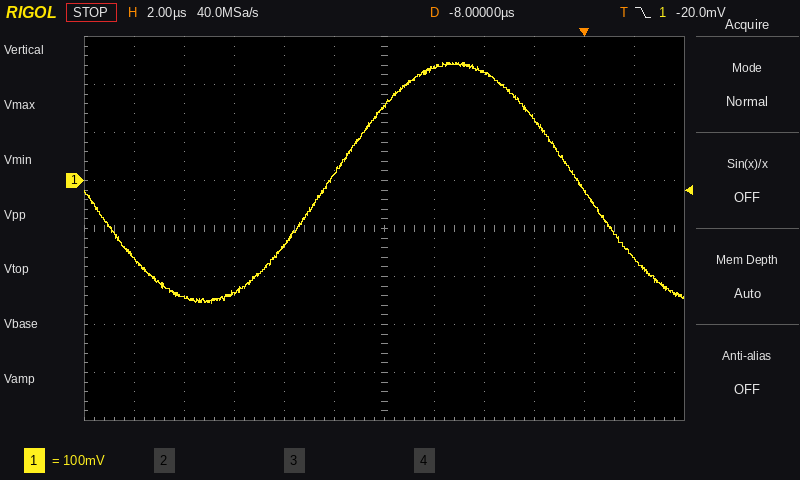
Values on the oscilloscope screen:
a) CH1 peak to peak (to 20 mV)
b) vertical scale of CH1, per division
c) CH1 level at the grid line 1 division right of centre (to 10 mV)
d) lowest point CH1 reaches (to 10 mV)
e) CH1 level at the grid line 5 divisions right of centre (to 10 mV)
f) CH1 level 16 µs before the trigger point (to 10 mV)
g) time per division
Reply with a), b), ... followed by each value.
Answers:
a) 500 mV
b) 100 mV
c) 240 mV
d) -260 mV
e) -160 mV
f) -240 mV
g) 2 µs
